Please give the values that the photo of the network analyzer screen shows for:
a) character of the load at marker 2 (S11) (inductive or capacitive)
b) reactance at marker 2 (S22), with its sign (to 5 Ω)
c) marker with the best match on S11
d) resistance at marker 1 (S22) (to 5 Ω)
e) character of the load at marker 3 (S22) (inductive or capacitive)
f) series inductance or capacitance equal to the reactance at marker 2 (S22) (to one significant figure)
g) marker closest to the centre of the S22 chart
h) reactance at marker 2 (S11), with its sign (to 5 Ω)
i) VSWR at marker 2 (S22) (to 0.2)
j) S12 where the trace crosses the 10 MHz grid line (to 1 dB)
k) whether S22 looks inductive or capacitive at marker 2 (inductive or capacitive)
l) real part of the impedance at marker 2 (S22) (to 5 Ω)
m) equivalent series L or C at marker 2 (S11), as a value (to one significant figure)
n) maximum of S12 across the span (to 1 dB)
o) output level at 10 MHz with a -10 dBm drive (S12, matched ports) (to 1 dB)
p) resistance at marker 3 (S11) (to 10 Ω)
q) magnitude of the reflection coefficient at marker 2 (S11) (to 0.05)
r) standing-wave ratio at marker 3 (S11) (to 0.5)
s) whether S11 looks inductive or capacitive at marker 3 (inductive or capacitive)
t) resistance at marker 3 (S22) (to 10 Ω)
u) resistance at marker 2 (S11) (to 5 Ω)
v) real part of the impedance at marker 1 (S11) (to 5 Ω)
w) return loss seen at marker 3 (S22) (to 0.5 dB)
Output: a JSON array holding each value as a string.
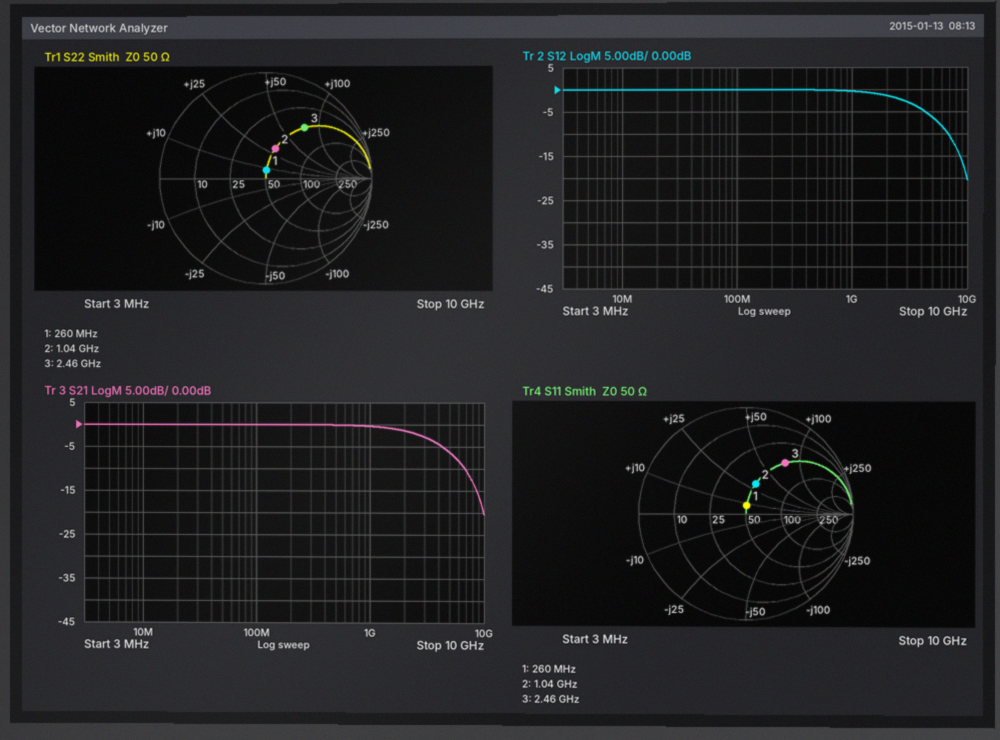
["inductive", "+30 Ω", "marker 1", "50 Ω", "inductive", "5 nH", "marker 1", "+30 Ω", "1.8", "0 dB", "inductive", "50 Ω", "5 nH", "0 dB", "-10 dBm", "50 Ω", "0.30", "4.0", "inductive", "50 Ω", "50 Ω", "50 Ω", "4.5 dB"]
